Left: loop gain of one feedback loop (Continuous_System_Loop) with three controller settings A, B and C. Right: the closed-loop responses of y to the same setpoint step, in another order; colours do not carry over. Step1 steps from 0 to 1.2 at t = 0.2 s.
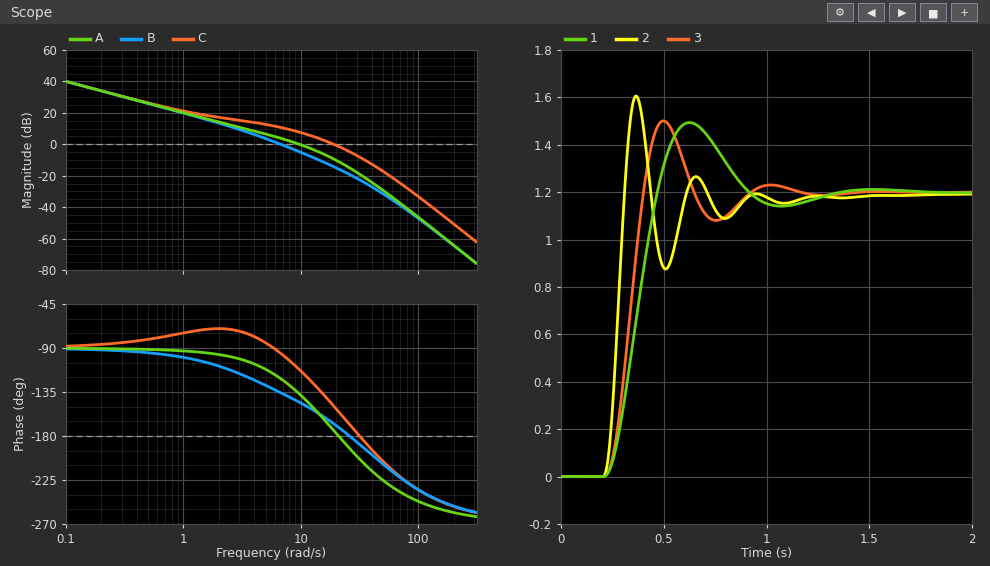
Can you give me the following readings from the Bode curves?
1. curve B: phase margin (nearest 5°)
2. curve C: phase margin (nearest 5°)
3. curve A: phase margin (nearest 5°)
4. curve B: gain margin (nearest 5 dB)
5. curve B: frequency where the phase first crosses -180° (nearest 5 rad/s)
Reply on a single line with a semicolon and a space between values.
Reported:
45°; 30°; 45°; 20 dB; 25 rad/s
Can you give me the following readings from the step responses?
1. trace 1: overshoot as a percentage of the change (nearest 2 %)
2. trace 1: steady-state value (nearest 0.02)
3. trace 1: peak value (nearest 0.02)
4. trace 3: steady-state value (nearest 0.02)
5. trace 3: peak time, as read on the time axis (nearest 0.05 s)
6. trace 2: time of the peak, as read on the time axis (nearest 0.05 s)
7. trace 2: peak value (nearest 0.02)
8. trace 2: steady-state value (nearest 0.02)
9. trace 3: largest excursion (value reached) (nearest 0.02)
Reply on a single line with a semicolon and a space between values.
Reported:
24 %; 1.20; 1.50; 1.20; 0.50 s; 0.35 s; 1.60; 1.20; 1.50
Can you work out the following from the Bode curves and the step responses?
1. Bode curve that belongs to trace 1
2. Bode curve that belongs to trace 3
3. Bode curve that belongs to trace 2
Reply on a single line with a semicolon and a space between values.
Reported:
B; A; C
